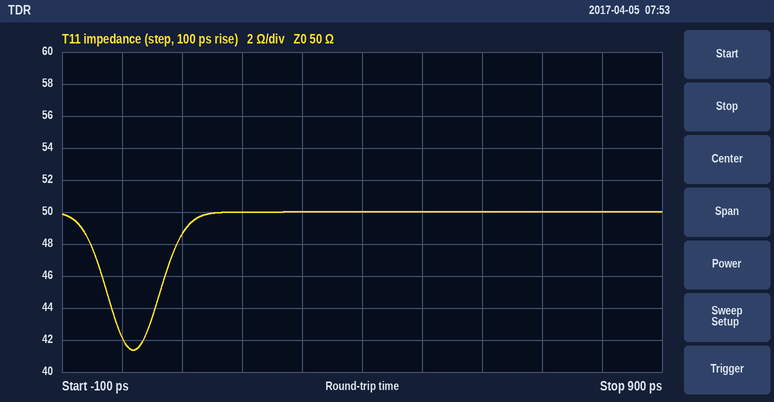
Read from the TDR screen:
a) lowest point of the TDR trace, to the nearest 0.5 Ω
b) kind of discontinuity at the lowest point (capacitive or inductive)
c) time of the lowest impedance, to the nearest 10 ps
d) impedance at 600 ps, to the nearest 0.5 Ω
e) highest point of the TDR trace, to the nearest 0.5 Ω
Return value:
41.5 Ω
capacitive
20 ps
50.0 Ω
50.0 Ω
